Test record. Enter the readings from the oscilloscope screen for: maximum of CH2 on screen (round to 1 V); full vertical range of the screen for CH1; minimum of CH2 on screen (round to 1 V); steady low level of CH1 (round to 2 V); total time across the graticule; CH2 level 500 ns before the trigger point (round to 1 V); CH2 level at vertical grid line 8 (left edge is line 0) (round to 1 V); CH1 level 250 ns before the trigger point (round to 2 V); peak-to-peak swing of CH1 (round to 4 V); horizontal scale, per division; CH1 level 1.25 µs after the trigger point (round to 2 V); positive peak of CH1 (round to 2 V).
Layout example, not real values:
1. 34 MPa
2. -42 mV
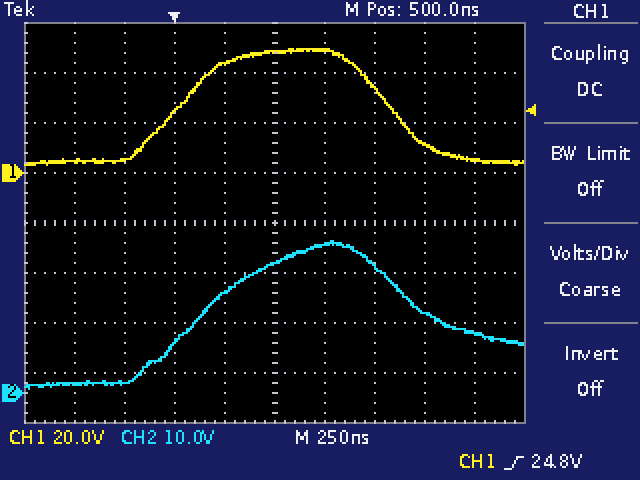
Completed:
1. 30 V
2. 160 V
3. 1 V
4. 4 V
5. 2.5 µs
6. 2 V
7. 16 V
8. 6 V
9. 48 V
10. 250 ns
11. 12 V
12. 50 V
